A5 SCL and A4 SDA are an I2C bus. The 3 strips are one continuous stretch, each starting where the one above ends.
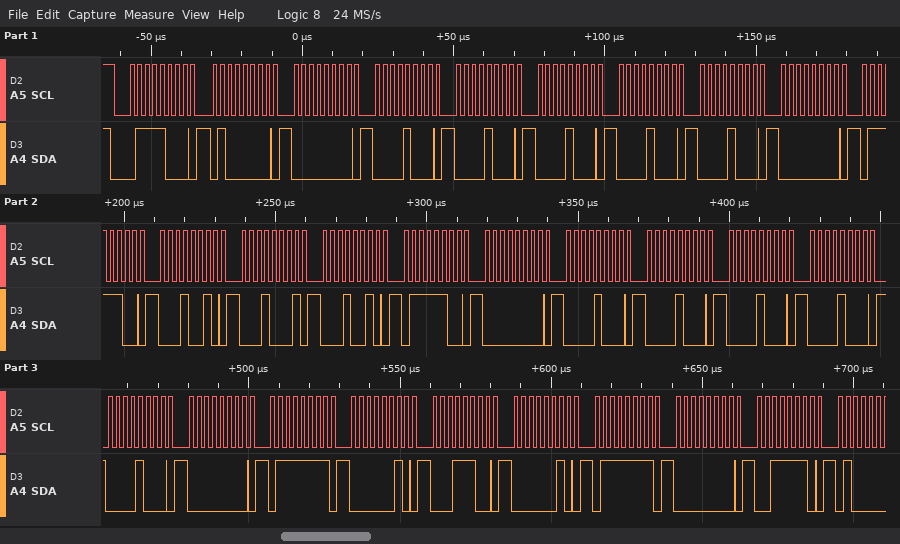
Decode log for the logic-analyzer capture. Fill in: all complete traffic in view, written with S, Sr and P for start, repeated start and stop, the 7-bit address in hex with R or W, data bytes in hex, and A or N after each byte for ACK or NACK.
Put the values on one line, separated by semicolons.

S 3CW A 40 A 00 A 08 A 08 A 08 A 08 A 08 A 00 A 7C A 12 A 11 A 12 A 7C A 00 A 08 A 08 A 08 A 08 A 08 A 00 A 7F A 02 A 1C A 02 A 7F A 00 A 3E A
